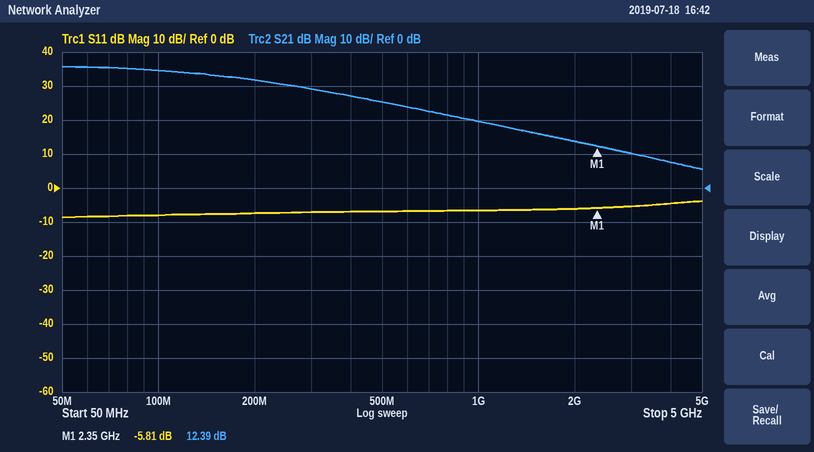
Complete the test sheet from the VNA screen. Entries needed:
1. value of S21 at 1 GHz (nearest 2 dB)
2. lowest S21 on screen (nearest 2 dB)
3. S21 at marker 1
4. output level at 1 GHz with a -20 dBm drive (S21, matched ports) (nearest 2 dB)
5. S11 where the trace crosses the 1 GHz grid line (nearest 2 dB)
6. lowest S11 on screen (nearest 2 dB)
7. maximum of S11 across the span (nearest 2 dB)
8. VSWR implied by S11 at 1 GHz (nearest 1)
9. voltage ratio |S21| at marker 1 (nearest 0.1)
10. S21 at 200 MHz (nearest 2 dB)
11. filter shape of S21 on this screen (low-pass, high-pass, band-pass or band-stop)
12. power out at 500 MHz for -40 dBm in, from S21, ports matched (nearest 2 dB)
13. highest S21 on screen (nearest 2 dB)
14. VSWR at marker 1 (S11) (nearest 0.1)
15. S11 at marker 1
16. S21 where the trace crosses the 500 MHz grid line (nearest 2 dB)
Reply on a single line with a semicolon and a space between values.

20 dB; 6 dB; 12.39 dB; 0 dBm; -6 dB; -8 dB; -4 dB; 3; 4.2; 32 dB; low-pass; -14 dBm; 36 dB; 3.1; -5.81 dB; 26 dB
